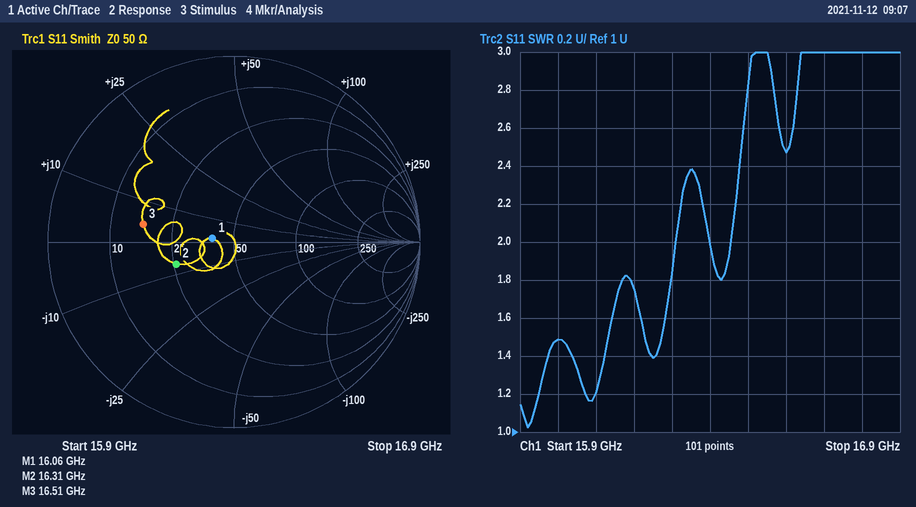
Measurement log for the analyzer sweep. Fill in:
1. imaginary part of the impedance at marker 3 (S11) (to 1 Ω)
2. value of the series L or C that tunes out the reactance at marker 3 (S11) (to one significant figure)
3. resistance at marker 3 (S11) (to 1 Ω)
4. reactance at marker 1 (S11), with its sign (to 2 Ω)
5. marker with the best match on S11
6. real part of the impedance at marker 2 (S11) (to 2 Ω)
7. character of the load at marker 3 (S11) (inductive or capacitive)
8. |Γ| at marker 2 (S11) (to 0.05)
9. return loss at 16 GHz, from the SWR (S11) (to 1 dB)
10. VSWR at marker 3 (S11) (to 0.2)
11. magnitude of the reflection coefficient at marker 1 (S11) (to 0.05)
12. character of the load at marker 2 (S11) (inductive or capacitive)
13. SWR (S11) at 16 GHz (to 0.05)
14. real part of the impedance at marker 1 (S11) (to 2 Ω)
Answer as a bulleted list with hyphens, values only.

- +4 Ω
- 2 pF
- 17 Ω
- +2 Ω
- marker 1
- 26 Ω
- inductive
- 0.35
- 14 dB
- 3.0
- 0.10
- capacitive
- 1.50
- 40 Ω
